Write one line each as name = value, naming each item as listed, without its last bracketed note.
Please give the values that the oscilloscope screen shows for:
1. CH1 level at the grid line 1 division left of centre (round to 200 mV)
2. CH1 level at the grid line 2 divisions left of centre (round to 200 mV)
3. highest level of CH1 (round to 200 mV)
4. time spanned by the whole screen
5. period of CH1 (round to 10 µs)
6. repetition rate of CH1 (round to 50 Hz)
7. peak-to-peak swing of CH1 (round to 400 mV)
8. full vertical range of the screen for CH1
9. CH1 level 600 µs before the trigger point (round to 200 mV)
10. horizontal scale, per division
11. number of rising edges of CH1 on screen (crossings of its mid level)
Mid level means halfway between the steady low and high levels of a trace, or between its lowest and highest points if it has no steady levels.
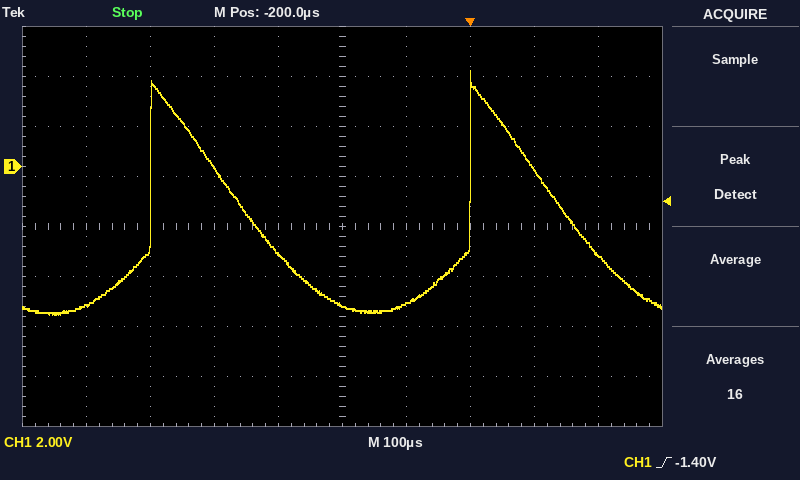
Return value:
CH1 level at the grid line 1 division left of centre = -3.4 V
CH1 level at the grid line 2 divisions left of centre = 0.0 V
highest level of CH1 = 3.8 V
time spanned by the whole screen = 1 ms
period of CH1 = 500 µs
repetition rate of CH1 = 2.00 kHz
peak-to-peak swing of CH1 = 9.6 V
full vertical range of the screen for CH1 = 16 V
CH1 level 600 µs before the trigger point = -5.6 V
horizontal scale, per division = 100 µs
number of rising edges of CH1 on screen = 2
